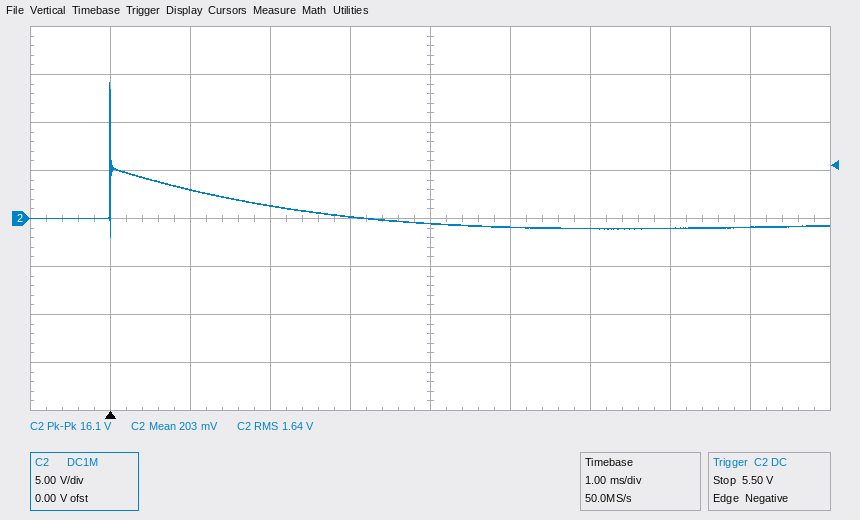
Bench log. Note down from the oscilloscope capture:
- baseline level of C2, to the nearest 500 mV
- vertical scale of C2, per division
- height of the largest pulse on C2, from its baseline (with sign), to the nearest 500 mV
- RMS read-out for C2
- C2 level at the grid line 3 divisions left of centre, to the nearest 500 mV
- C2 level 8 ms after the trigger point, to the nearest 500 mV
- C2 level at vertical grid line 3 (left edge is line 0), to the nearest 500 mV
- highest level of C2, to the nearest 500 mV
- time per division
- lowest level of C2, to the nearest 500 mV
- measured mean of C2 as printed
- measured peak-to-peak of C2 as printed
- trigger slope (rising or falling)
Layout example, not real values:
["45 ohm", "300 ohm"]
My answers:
["-1.0 V", "5 V", "+15.0 V", "1.64 V", "3.0 V", "-1.0 V", "1.5 V", "14.0 V", "1 ms", "-2.0 V", "203 mV", "16.1 V", "falling"]
